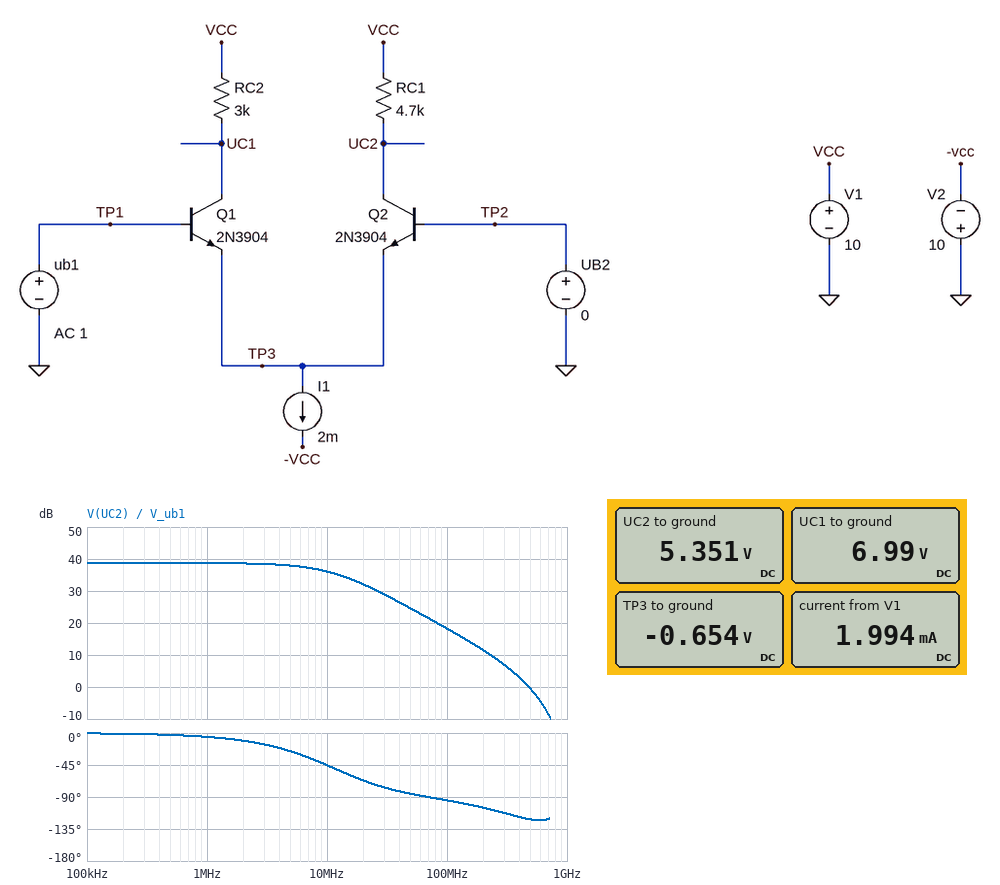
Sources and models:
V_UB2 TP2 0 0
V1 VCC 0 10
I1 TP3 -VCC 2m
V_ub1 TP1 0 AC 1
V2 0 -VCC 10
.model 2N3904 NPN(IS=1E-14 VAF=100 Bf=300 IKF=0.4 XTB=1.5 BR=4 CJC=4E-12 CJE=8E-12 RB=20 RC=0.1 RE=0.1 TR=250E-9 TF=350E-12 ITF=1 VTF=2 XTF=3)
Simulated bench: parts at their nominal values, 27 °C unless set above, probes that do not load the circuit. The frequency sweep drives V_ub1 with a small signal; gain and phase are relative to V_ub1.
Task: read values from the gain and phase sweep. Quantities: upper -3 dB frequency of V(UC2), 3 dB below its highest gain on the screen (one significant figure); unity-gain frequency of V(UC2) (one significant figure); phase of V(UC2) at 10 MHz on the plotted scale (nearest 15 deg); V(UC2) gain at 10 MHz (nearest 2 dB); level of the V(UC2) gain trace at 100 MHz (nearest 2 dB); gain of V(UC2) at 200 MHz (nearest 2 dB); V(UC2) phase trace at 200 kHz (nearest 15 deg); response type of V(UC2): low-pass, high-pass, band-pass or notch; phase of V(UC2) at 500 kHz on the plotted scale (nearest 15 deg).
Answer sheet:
10 MHz
500 MHz
-45 deg
36 dB
18 dB
12 dB
0 deg
low-pass
0 deg
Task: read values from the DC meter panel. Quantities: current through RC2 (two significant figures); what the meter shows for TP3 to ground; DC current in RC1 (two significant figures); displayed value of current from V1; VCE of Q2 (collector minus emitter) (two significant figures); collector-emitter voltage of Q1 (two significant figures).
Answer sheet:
1.0 mA
-0.654 V
990 µA
1.994 mA
6.0 V
7.6 V
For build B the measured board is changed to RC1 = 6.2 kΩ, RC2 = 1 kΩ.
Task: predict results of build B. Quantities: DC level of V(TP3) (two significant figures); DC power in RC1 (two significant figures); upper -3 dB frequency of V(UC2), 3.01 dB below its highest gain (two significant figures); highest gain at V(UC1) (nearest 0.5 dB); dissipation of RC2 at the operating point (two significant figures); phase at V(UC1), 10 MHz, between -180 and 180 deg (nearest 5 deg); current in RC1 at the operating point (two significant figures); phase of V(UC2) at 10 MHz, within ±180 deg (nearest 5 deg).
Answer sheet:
-650 mV
5.9 mW
8.5 MHz
25.5 dB
1.0 mW
160 deg
970 µA
-50 deg
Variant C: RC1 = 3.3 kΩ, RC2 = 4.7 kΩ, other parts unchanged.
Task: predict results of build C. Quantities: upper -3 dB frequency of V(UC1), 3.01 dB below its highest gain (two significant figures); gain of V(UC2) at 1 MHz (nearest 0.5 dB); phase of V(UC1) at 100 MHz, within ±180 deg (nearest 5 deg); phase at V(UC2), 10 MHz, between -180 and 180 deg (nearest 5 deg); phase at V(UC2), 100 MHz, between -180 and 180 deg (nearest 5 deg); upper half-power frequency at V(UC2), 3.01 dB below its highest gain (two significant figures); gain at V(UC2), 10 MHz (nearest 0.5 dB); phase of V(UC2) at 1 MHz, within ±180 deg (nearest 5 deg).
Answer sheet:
11 MHz
35.5 dB
80 deg
-35 deg
-90 deg
13 MHz
33.5 dB
-5 deg
